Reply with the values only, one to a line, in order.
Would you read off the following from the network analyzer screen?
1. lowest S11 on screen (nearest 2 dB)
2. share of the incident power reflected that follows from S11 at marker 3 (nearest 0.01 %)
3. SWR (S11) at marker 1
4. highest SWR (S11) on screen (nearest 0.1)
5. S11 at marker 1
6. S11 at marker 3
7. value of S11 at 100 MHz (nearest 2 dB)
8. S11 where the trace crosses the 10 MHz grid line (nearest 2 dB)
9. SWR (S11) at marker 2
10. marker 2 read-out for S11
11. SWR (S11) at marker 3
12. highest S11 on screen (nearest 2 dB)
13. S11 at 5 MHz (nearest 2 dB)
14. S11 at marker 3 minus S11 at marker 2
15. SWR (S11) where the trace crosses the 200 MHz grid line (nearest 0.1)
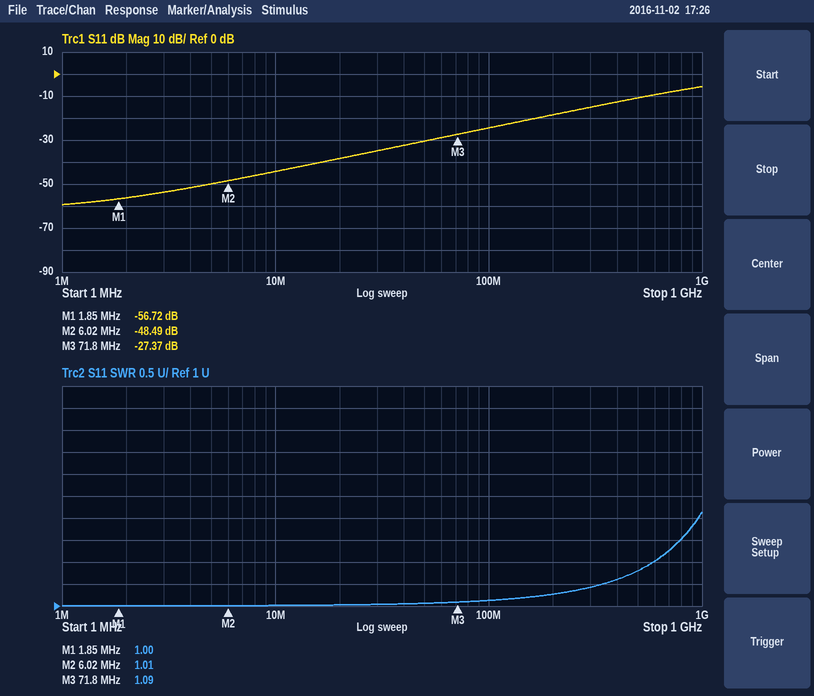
-60 dB
0.18 %
1.00
3.1
-56.72 dB
-27.37 dB
-24 dB
-44 dB
1.01
-48.49 dB
1.09
-6 dB
-50 dB
21.12 dB
1.3
